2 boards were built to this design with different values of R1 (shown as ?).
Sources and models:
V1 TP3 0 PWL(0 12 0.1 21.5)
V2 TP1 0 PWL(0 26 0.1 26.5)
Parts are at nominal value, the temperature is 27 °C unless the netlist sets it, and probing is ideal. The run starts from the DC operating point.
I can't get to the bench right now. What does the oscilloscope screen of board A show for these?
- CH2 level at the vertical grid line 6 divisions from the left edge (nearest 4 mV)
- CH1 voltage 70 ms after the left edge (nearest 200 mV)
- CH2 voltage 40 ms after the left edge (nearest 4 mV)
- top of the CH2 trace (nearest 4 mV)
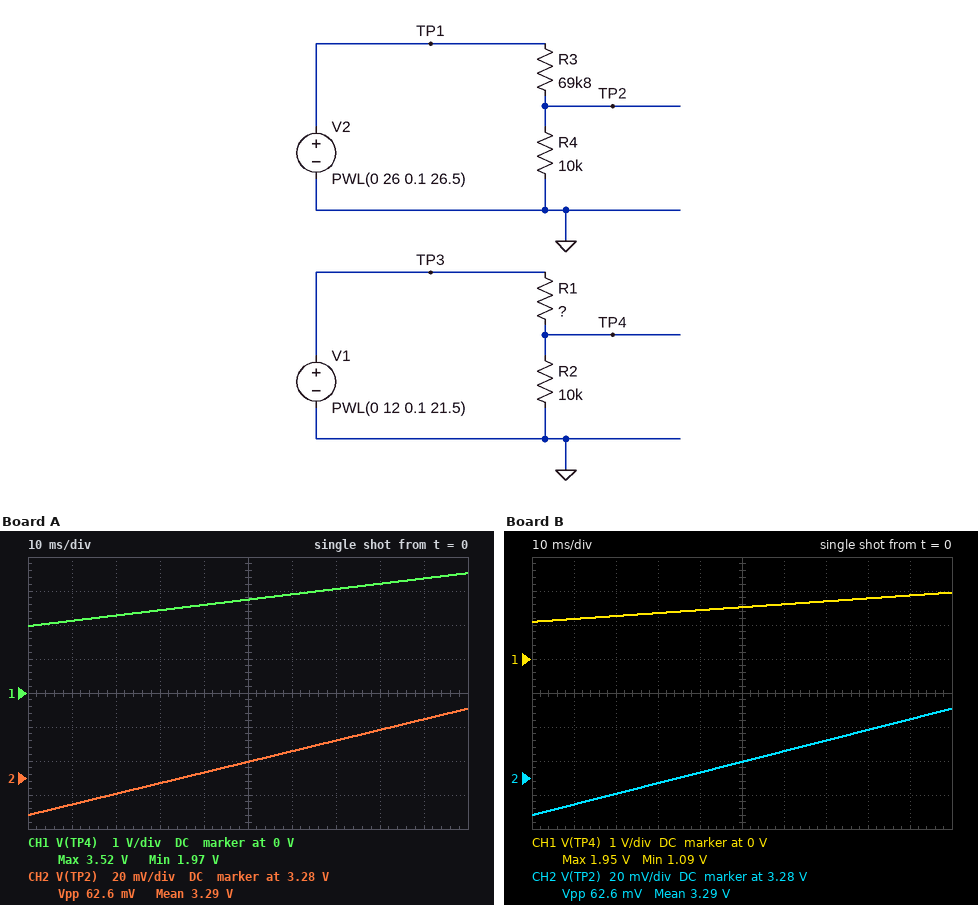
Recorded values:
3.296 V
3.0 V
3.284 V
3.320 V
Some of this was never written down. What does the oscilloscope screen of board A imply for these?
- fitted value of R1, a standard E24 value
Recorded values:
51 kΩ
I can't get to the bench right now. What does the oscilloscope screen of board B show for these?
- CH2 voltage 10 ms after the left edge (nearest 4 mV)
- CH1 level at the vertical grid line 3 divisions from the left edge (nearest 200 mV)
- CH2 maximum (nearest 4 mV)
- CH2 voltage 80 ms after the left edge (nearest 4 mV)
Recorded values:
3.264 V
1.4 V
3.320 V
3.308 V
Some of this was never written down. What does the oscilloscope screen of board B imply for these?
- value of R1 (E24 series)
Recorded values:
100 kΩ
